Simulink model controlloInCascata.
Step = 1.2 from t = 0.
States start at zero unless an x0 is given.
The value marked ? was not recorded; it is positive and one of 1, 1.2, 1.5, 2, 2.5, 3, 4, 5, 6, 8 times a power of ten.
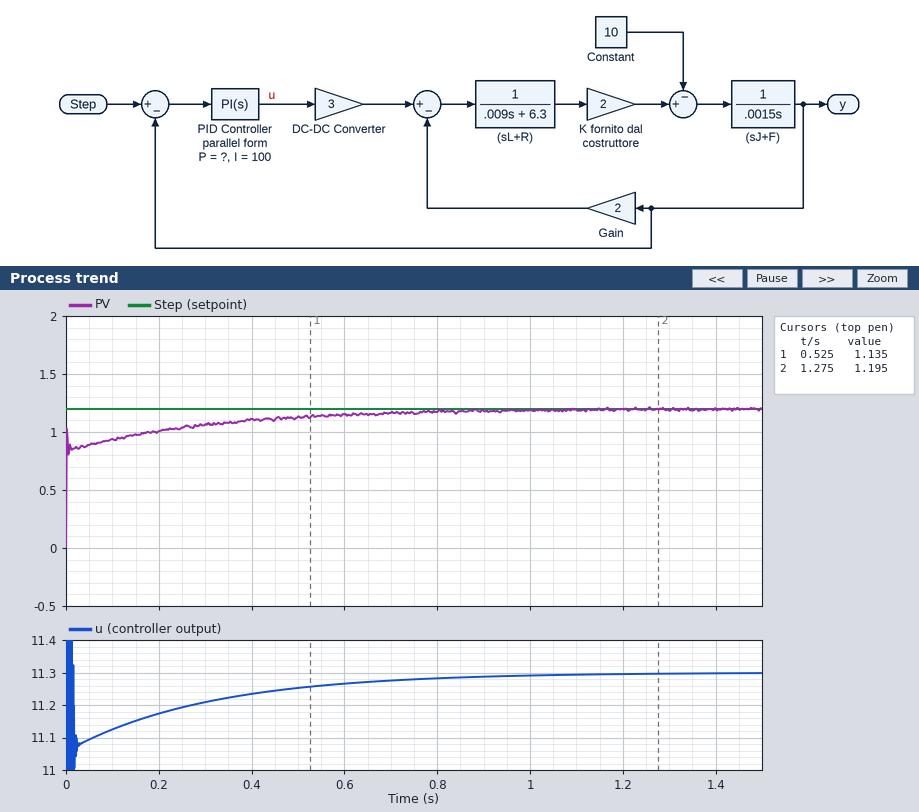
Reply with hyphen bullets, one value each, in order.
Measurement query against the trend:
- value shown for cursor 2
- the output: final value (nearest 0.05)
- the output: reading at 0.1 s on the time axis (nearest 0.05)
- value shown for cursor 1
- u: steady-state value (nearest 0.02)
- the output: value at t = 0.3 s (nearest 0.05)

- 1.195
- 1.20
- 0.95
- 1.135
- 11.30
- 1.05
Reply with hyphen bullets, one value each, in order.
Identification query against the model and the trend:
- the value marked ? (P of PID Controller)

- 30
